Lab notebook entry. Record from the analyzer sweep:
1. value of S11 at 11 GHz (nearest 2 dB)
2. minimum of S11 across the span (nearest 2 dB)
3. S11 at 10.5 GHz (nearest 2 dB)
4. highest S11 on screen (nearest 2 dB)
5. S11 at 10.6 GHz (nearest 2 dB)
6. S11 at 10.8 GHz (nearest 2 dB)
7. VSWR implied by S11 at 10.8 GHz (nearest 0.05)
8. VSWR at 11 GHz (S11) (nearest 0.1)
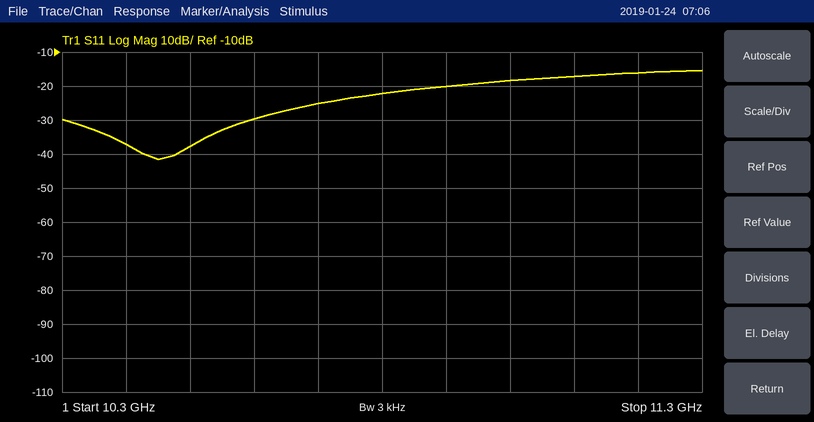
-18 dB
-42 dB
-38 dB
-16 dB
-30 dB
-22 dB
1.15
1.3
